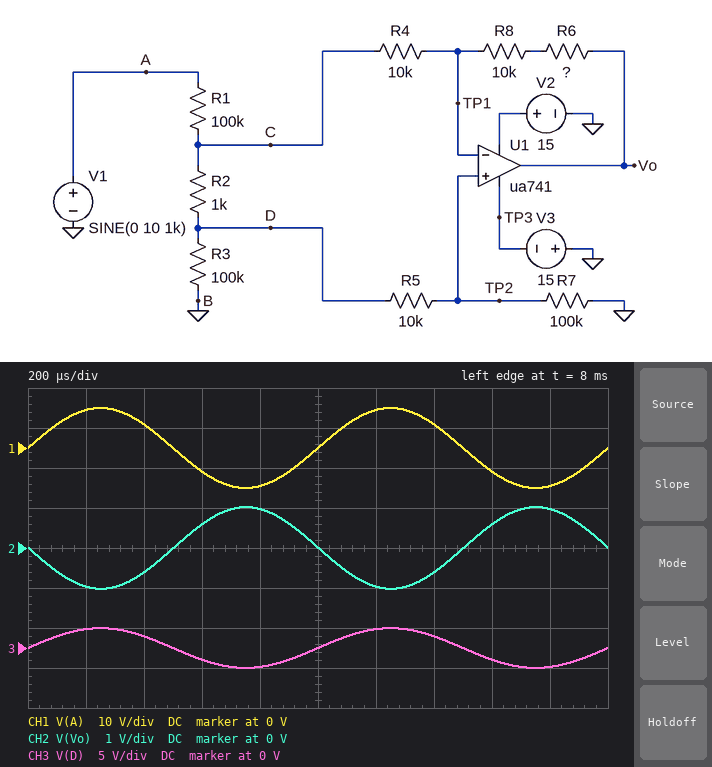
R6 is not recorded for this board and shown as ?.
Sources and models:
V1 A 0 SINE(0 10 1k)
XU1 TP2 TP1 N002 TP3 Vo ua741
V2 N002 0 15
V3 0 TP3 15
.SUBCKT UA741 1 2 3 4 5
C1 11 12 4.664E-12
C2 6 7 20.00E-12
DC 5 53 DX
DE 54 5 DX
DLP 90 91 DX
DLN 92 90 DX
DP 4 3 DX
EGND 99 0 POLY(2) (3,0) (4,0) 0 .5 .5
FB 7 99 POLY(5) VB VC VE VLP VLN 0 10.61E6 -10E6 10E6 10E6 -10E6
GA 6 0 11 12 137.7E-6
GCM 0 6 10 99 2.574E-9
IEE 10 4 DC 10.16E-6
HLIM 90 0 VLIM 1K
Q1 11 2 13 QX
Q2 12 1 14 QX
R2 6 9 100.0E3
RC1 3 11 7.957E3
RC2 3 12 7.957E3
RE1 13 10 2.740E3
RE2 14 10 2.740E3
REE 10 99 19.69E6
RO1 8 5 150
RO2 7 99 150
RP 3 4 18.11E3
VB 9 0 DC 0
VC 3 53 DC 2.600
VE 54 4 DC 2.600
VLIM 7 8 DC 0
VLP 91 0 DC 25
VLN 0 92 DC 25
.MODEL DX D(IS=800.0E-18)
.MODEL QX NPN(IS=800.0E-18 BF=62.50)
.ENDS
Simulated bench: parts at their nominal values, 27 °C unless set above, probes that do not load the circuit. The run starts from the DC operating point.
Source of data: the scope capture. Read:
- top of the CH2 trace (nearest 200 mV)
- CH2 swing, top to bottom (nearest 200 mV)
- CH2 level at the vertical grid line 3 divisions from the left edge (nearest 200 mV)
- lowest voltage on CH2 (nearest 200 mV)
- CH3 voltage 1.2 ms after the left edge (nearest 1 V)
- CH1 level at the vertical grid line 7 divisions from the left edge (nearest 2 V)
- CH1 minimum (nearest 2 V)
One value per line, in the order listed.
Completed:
1.0 V
2.0 V
600 mV
-1.0 V
2 V
6 V
-10 V
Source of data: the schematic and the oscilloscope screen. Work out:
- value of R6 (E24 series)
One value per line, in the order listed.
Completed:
110 kΩ
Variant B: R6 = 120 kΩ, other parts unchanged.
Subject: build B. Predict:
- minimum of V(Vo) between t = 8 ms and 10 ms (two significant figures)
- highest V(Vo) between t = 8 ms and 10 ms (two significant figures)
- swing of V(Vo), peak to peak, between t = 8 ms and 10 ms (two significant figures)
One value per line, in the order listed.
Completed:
-1.3 V
1.3 V
2.6 V
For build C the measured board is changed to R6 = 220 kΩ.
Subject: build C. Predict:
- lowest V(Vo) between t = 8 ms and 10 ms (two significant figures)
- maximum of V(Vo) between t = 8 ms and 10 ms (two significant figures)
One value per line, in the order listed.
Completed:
-4.0 V
4.0 V
